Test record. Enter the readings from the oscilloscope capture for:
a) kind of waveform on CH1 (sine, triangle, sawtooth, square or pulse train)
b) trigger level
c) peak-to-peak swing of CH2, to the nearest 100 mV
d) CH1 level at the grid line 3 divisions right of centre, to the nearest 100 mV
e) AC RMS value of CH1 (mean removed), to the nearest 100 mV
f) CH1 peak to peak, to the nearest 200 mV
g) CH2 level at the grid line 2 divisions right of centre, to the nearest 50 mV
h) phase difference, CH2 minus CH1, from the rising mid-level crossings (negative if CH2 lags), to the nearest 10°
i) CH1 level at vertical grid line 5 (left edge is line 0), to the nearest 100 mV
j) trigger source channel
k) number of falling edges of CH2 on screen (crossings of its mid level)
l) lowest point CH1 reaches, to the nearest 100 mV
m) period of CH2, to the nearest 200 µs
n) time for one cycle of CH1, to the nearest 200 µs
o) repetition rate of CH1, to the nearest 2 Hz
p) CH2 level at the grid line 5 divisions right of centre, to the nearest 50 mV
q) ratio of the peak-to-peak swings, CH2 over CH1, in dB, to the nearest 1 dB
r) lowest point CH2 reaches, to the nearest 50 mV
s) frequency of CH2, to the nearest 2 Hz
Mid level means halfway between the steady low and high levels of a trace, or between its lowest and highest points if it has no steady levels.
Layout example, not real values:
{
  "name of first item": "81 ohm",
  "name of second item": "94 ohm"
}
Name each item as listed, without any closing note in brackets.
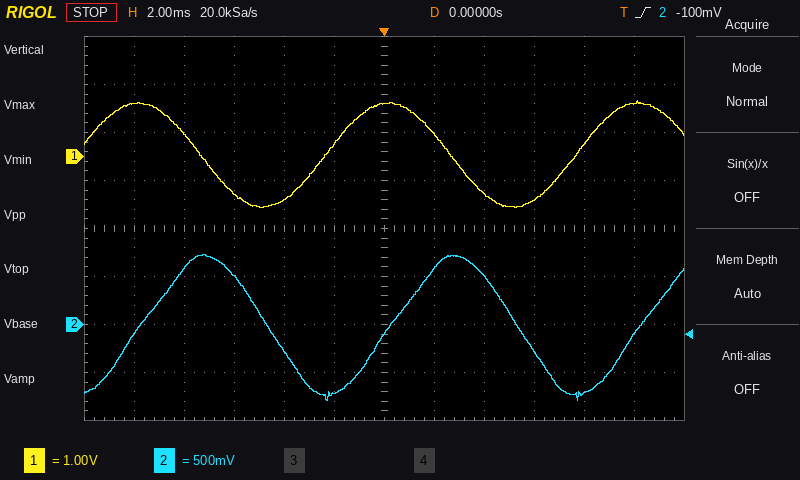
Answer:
{
  "kind of waveform on CH1": "sine",
  "trigger level": "-100 mV",
  "peak-to-peak swing of CH2, to the nearest 100 mV": "1.50 V",
  "CH1 level at the grid line 3 divisions right of centre, to the nearest 100 mV": "-900 mV",
  "AC RMS value of CH1 (mean removed), to the nearest 100 mV": "800 mV",
  "CH1 peak to peak, to the nearest 200 mV": "2.2 V",
  "CH2 level at the grid line 2 divisions right of centre, to the nearest 50 mV": "500 mV",
  "phase difference, CH2 minus CH1, from the rising mid-level crossings (negative if CH2 lags), to the nearest 10°": "-90°",
  "CH1 level at vertical grid line 5 (left edge is line 0), to the nearest 100 mV": "300 mV",
  "trigger source channel": "CH2",
  "number of falling edges of CH2 on screen": "2",
  "lowest point CH1 reaches, to the nearest 100 mV": "-1.1 V",
  "period of CH2, to the nearest 200 µs": "10.0 ms",
  "time for one cycle of CH1, to the nearest 200 µs": "10.0 ms",
  "repetition rate of CH1, to the nearest 2 Hz": "100 Hz",
  "CH2 level at the grid line 5 divisions right of centre, to the nearest 50 mV": "-100 mV",
  "ratio of the peak-to-peak swings, CH2 over CH1, in dB, to the nearest 1 dB": "-3 dB",
  "lowest point CH2 reaches, to the nearest 50 mV": "-800 mV",
  "frequency of CH2, to the nearest 2 Hz": "100 Hz"
}
